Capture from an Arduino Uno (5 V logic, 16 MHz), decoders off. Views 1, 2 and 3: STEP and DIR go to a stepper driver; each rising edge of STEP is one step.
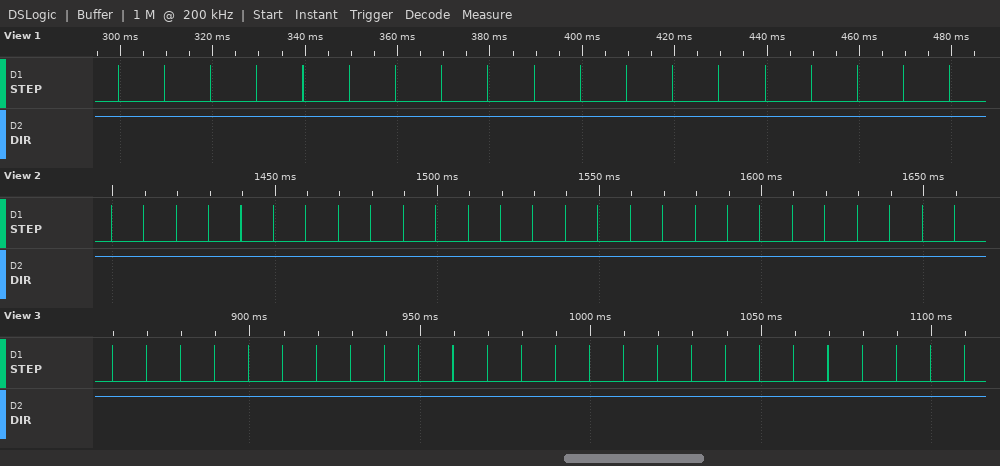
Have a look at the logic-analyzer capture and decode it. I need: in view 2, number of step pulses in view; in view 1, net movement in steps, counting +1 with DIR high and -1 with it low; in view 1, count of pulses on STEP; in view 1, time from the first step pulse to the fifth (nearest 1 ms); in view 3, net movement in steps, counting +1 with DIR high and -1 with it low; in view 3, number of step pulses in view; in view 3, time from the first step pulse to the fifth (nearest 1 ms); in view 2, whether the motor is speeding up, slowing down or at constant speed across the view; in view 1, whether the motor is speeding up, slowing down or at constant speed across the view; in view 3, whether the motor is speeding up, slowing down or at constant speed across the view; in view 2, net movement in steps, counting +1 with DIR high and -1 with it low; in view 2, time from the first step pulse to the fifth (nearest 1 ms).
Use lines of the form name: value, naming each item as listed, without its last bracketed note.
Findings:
in view 2, number of step pulses in view: 27
in view 1, net movement in steps, counting +1 with DIR high and -1 with it low: +19
in view 1, count of pulses on STEP: 19
in view 1, time from the first step pulse to the fifth: 40 ms
in view 3, net movement in steps, counting +1 with DIR high and -1 with it low: +26
in view 3, number of step pulses in view: 26
in view 3, time from the first step pulse to the fifth: 40 ms
in view 2, whether the motor is speeding up, slowing down or at constant speed across the view: constant speed
in view 1, whether the motor is speeding up, slowing down or at constant speed across the view: constant speed
in view 3, whether the motor is speeding up, slowing down or at constant speed across the view: constant speed
in view 2, net movement in steps, counting +1 with DIR high and -1 with it low: +27
in view 2, time from the first step pulse to the fifth: 40 ms
